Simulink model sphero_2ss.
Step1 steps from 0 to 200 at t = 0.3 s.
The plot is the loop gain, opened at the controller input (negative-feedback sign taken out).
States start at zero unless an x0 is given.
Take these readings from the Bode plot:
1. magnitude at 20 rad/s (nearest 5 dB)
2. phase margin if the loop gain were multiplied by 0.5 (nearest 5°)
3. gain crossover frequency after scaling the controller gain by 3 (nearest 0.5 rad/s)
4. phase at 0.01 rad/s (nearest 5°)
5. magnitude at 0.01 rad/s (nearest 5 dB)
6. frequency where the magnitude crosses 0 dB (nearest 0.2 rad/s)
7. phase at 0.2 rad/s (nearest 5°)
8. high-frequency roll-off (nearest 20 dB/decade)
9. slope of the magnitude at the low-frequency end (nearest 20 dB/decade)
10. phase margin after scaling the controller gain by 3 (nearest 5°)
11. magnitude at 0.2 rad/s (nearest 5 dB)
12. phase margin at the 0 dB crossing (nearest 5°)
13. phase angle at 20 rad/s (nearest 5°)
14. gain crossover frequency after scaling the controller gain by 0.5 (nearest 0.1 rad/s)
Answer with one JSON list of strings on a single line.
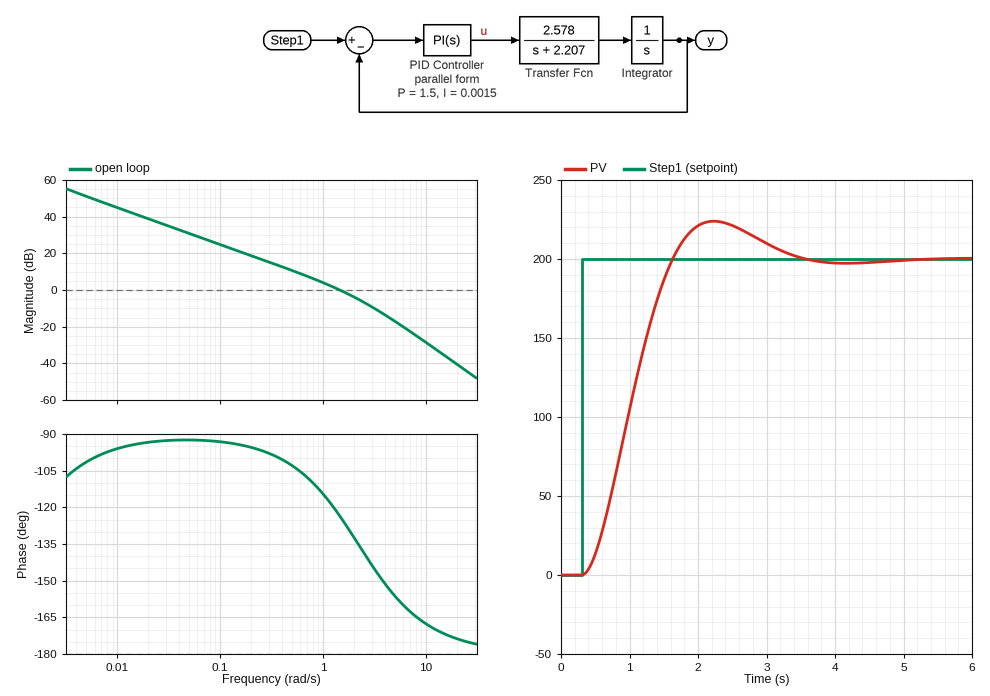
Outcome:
["-40 dB", "70°", "3.0 rad/s", "-95°", "45 dB", "1.4 rad/s", "-95°", "-40 dB/decade", "-20 dB/decade", "35°", "20 dB", "55°", "-175°", "0.8 rad/s"]
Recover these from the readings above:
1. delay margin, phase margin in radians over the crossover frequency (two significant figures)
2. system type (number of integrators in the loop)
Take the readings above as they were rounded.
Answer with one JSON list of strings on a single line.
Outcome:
["0.69 s", "1"]
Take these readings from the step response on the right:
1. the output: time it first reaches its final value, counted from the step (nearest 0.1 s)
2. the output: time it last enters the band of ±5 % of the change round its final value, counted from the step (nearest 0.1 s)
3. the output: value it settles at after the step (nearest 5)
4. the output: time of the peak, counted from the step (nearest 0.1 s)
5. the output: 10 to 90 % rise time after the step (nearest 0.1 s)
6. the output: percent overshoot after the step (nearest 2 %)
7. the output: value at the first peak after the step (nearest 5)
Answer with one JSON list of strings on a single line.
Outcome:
["1.3 s", "2.7 s", "200", "1.9 s", "0.9 s", "12 %", "225"]
